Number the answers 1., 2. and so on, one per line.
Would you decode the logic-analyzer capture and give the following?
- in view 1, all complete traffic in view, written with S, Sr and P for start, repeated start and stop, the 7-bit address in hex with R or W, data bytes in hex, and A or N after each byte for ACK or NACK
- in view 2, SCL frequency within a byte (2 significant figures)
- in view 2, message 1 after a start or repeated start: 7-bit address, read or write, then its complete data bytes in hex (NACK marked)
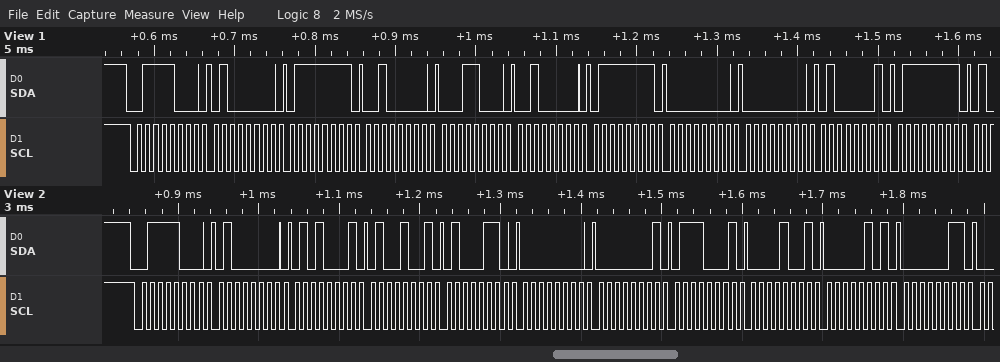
1. S 3CW A 40 A 7F A 20 A 18 A 20 A 7F A 00 A 00 A 41 A 7F A
2. 100 kHz
3. 0x3C write: 40 51 49 46 00 01 71 09 05 03
